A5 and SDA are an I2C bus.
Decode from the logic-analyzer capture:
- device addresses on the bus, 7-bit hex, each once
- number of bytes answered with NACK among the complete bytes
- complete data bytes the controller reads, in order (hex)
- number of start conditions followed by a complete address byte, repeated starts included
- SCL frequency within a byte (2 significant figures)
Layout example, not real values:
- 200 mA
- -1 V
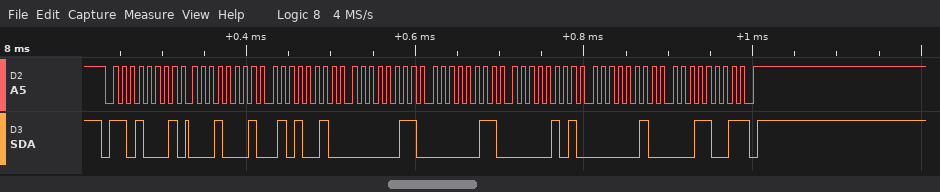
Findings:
- 0x68
- 1
- 11 52 03 03 05 02 19
- 1
- 100 kHz
